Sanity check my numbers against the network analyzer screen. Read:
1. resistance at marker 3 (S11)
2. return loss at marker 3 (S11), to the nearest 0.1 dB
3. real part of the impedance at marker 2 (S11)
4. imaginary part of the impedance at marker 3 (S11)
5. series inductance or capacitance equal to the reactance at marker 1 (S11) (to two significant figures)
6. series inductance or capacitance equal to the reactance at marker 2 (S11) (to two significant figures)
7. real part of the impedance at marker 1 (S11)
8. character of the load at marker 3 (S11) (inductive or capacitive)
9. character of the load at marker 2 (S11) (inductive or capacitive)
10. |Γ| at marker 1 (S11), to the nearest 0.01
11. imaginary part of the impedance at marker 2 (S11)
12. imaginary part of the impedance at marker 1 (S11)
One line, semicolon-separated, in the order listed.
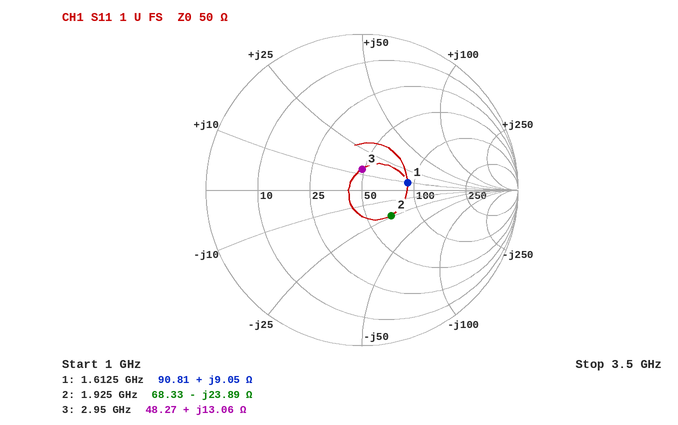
48.27 Ω; 17.5 dB; 68.33 Ω; +13.06 Ω; 890 pH; 3.5 pF; 90.81 Ω; inductive; capacitive; 0.30; -23.89 Ω; +9.05 Ω
